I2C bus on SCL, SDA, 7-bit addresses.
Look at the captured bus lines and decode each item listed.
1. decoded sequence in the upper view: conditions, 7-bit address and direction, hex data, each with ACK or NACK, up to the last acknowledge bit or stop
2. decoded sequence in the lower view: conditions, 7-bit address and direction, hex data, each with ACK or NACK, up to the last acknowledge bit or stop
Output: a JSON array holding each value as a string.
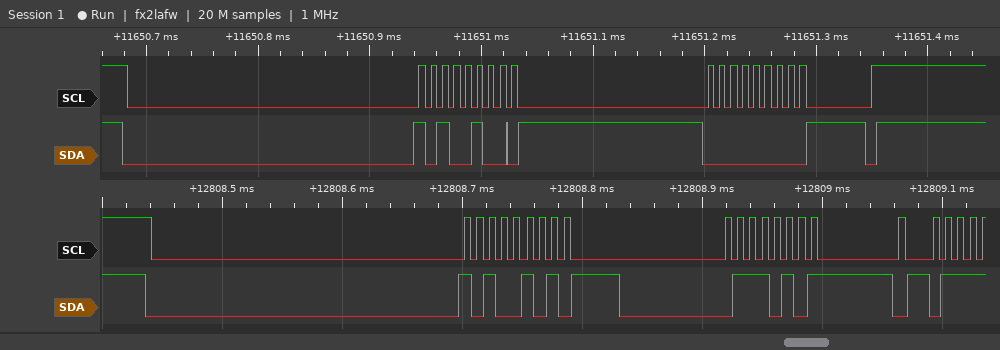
["start, address 52 write ACK, 00 ACK, stop", "start, address 52 read ACK, 75 ACK"]
